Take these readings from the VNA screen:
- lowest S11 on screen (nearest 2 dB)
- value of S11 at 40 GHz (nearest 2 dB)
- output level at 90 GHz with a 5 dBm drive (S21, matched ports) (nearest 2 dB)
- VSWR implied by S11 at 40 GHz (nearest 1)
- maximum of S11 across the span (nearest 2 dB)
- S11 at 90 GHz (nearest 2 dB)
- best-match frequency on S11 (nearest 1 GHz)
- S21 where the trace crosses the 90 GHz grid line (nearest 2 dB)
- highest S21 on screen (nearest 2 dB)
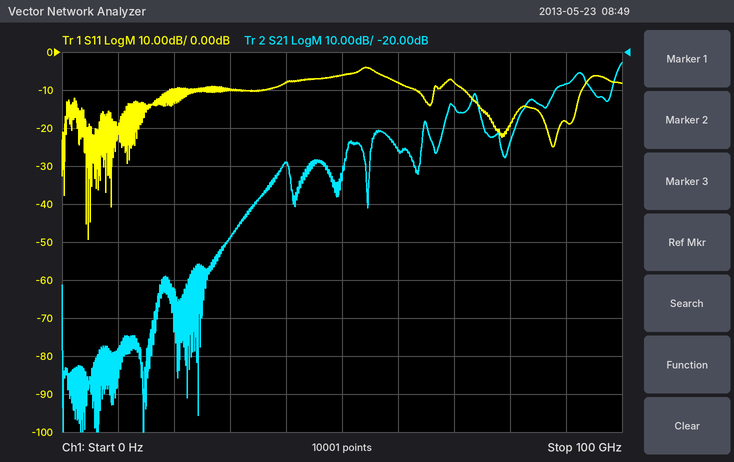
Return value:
-50 dB
-8 dB
-24 dBm
2
-4 dB
-18 dB
5 GHz
-28 dB
-22 dB
